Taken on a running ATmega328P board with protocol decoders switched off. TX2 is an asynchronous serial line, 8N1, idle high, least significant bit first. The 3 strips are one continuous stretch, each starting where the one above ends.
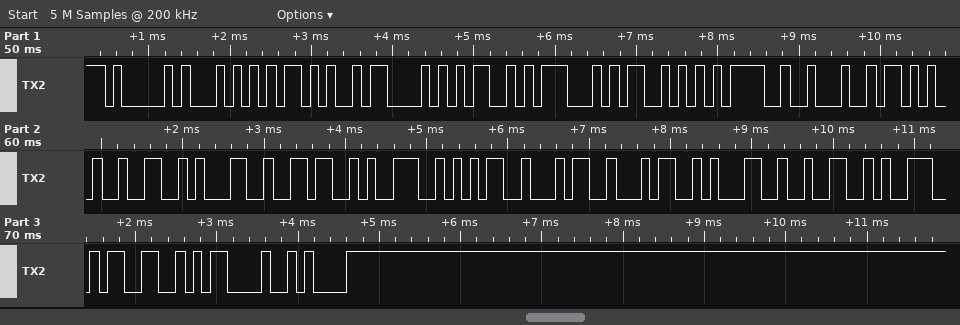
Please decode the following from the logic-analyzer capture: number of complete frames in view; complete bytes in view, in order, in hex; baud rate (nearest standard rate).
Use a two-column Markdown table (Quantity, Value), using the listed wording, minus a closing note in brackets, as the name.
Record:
| Quantity | Value |
|---|---|
| number of complete frames in view | 23 |
| complete bytes in view, in order, in hex | 41 54 2B 43 4D 47 53 3D 22 2B 32 31 36 39 35 34 34 31 32 39 33 0D 0A |
| baud rate | 9600 baud |
